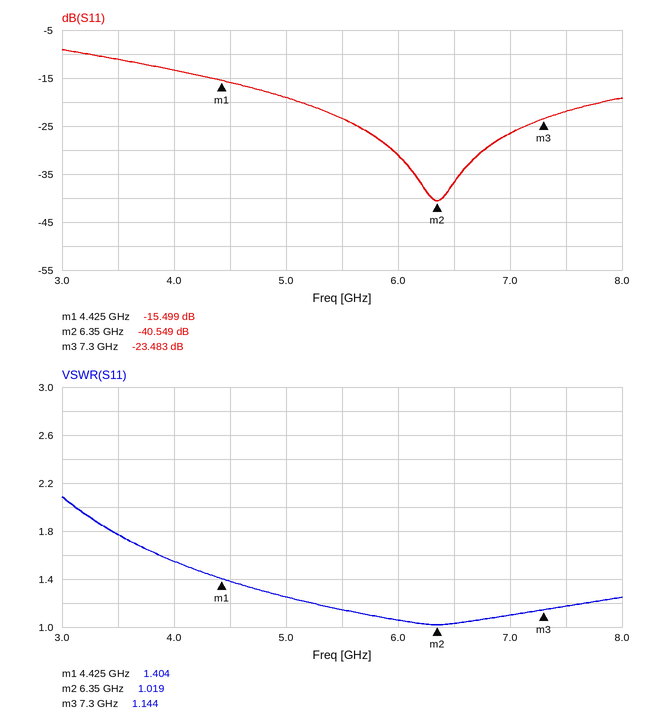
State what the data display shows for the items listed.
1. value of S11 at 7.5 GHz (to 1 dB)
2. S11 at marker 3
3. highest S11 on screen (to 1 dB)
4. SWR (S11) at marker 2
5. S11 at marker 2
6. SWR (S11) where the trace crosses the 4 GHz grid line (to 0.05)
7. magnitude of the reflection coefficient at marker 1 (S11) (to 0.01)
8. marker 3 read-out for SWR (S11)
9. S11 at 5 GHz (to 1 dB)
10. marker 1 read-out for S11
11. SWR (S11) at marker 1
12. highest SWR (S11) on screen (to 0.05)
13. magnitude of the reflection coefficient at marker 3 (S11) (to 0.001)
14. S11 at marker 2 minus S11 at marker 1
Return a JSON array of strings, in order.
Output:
["-22 dB", "-23.483 dB", "-9 dB", "1.019", "-40.549 dB", "1.55", "0.17", "1.144", "-19 dB", "-15.499 dB", "1.404", "2.10", "0.067", "-25.050 dB"]
